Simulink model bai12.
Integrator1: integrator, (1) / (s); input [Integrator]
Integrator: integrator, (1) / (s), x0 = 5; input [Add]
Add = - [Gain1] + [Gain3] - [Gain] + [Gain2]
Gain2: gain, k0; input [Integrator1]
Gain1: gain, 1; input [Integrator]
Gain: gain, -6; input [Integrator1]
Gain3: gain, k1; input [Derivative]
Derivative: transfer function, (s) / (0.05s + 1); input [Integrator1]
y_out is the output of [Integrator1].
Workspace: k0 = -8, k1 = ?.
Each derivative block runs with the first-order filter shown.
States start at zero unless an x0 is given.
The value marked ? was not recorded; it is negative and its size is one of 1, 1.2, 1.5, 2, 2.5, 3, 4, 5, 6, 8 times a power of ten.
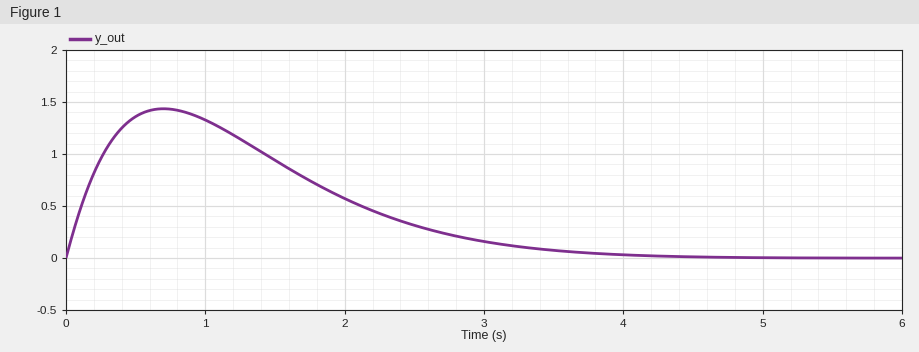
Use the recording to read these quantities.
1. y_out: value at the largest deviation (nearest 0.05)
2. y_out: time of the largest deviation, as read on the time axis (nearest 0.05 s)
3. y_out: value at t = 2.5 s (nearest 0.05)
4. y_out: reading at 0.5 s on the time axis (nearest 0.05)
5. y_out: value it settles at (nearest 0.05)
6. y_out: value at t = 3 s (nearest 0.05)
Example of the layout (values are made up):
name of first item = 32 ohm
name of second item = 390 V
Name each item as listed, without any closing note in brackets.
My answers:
y_out: value at the largest deviation = 1.45
y_out: time of the largest deviation, as read on the time axis = 0.70 s
y_out: value at t = 2.5 s = 0.30
y_out: reading at 0.5 s on the time axis = 1.35
y_out: value it settles at = 0.00
y_out: value at t = 3 s = 0.15
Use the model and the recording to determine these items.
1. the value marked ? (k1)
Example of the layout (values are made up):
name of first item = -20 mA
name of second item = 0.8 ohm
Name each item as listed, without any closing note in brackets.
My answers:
the value marked ? = -1.5
